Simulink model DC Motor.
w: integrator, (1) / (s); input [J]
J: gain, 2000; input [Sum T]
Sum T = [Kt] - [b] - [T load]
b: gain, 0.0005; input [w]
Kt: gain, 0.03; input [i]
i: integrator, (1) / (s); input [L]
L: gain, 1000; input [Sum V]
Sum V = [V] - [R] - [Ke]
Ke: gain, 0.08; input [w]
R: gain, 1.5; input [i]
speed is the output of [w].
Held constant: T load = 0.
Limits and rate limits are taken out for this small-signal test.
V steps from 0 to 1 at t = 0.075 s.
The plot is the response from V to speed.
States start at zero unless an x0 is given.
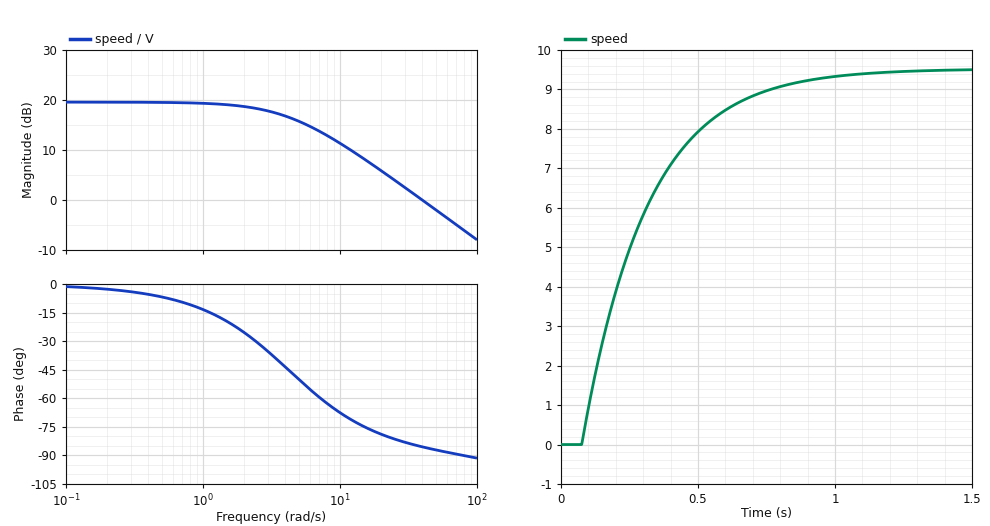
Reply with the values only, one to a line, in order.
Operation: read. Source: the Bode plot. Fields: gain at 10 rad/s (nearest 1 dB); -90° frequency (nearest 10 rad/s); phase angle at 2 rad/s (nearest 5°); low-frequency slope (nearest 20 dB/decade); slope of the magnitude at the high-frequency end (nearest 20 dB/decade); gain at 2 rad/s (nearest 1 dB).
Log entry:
11 dB
80 rad/s
-25°
0 dB/decade
-20 dB/decade
19 dB
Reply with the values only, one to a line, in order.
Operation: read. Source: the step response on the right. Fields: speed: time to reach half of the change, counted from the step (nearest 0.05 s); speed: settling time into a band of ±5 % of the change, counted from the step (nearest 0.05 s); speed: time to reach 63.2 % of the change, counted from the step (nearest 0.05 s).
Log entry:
0.15 s
0.70 s
0.25 s
